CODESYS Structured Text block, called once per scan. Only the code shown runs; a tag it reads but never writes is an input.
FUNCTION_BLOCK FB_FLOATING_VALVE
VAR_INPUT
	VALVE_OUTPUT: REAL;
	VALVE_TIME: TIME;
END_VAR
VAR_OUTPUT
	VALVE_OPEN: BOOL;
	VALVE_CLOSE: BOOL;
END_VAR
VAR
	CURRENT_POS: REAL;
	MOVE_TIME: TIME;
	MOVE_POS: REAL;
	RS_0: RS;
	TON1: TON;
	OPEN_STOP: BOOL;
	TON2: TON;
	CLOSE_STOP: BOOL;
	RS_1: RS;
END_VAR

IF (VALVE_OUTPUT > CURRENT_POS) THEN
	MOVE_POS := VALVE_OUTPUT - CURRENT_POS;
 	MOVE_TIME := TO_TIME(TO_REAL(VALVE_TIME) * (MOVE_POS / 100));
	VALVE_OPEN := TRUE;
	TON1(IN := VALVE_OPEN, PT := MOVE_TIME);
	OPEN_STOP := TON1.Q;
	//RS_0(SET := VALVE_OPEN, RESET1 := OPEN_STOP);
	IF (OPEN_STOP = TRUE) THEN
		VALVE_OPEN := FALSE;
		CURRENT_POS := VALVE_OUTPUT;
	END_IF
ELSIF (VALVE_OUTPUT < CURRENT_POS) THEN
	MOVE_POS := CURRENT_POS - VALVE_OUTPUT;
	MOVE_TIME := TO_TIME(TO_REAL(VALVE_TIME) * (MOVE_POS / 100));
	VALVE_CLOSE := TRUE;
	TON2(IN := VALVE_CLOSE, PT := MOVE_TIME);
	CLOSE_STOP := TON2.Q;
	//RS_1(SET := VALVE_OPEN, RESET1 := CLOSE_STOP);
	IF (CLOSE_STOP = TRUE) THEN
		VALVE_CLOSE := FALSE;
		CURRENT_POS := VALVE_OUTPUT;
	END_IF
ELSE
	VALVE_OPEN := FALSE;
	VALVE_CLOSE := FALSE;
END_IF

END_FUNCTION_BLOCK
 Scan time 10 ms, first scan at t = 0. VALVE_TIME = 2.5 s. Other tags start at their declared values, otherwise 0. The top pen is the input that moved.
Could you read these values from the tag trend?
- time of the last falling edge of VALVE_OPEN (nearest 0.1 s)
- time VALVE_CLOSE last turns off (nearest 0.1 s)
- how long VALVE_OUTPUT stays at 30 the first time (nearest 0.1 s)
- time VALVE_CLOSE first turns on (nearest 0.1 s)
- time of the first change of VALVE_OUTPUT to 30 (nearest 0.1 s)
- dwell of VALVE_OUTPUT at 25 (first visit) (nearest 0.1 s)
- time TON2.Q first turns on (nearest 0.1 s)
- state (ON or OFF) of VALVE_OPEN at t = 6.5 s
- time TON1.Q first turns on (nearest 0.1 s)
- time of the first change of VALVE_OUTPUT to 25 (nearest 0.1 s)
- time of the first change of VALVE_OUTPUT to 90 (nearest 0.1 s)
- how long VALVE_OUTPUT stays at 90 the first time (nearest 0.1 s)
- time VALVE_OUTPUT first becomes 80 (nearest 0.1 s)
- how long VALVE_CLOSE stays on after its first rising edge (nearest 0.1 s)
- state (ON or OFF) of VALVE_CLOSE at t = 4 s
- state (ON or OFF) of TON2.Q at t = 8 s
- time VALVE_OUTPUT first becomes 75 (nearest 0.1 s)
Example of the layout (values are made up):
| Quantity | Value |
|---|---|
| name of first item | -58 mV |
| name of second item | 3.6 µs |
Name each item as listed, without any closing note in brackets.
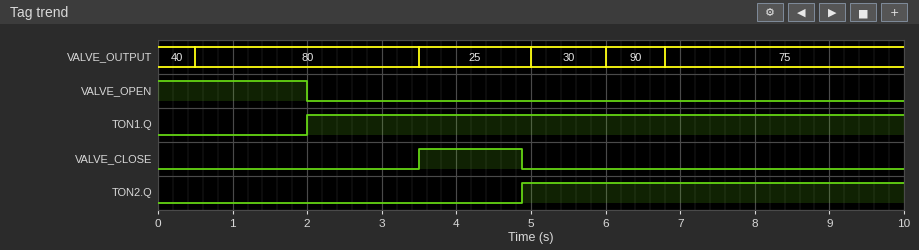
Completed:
| Quantity | Value |
|---|---|
| time of the last falling edge of VALVE_OPEN | 2.0 s |
| time VALVE_CLOSE last turns off | 4.9 s |
| how long VALVE_OUTPUT stays at 30 the first time | 1.0 s |
| time VALVE_CLOSE first turns on | 3.5 s |
| time of the first change of VALVE_OUTPUT to 30 | 5.0 s |
| dwell of VALVE_OUTPUT at 25 (first visit) | 1.5 s |
| time TON2.Q first turns on | 4.9 s |
| state (ON or OFF) of VALVE_OPEN at t = 6.5 s | OFF |
| time TON1.Q first turns on | 2.0 s |
| time of the first change of VALVE_OUTPUT to 25 | 3.5 s |
| time of the first change of VALVE_OUTPUT to 90 | 6.0 s |
| how long VALVE_OUTPUT stays at 90 the first time | 0.8 s |
| time VALVE_OUTPUT first becomes 80 | 0.5 s |
| how long VALVE_CLOSE stays on after its first rising edge | 1.4 s |
| state (ON or OFF) of VALVE_CLOSE at t = 4 s | ON |
| state (ON or OFF) of TON2.Q at t = 8 s | ON |
| time VALVE_OUTPUT first becomes 75 | 6.8 s |
